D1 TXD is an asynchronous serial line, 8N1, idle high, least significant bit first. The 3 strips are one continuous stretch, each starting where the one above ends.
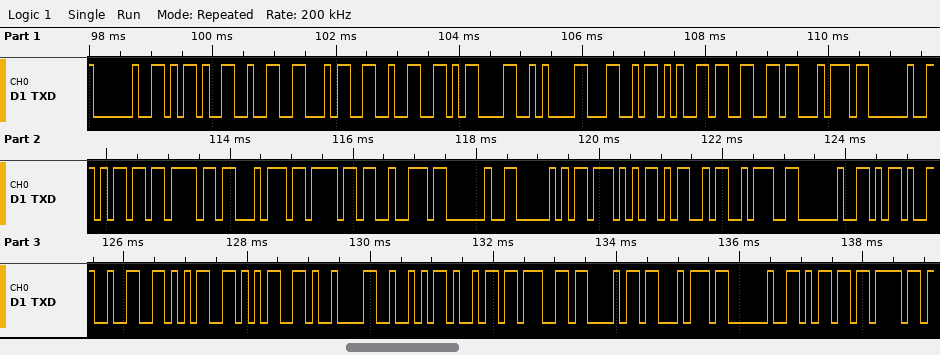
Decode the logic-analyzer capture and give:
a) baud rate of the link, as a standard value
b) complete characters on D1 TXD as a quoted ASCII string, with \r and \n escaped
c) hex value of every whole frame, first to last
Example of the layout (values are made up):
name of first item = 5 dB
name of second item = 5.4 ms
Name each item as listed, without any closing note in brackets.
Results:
baud rate of the link, as a standard value = 9600 baud
complete characters on D1 TXD as a quoted ASCII string, with \r and \n escaped = " -242\r\nLeft motor PWM: -255\tRight mo"
hex value of every whole frame, first to last = 0x20 0x2D 0x32 0x34 0x32 0x0D 0x0A 0x4C 0x65 0x66 0x74 0x20 0x6D 0x6F 0x74 0x6F 0x72 0x20 0x50 0x57 0x4D 0x3A 0x20 0x2D 0x32 0x35 0x35 0x09 0x52 0x69 0x67 0x68 0x74 0x20 0x6D 0x6F
